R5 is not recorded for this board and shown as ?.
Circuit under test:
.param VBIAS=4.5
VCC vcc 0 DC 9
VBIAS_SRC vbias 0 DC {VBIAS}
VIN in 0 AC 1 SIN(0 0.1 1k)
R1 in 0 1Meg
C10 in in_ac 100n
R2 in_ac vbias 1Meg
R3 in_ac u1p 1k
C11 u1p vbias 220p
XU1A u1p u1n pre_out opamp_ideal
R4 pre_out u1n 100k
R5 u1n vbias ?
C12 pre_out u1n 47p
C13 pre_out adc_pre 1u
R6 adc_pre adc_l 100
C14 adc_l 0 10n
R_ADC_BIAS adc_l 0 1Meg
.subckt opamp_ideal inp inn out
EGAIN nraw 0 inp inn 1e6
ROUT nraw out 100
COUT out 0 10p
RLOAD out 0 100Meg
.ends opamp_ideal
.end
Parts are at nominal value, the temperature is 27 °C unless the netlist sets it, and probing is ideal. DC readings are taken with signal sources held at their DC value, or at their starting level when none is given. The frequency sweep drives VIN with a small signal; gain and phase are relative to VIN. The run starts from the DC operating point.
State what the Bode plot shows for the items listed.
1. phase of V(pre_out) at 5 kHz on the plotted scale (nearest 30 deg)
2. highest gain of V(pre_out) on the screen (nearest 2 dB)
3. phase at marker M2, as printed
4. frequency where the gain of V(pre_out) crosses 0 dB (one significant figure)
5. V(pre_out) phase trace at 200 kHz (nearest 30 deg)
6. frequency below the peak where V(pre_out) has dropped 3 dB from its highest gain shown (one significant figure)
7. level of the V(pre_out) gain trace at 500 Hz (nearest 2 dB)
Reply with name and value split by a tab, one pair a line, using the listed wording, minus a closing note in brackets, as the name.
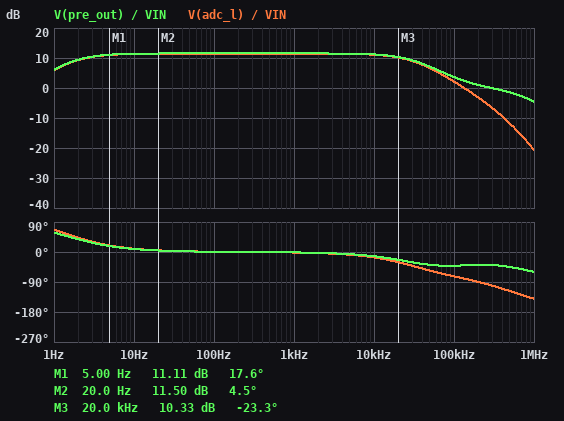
phase of V(pre_out) at 5 kHz on the plotted scale	0 deg
highest gain of V(pre_out) on the screen	12 dB
phase at marker M2, as printed	4.5 deg
frequency where the gain of V(pre_out) crosses 0 dB	300 kHz
V(pre_out) phase trace at 200 kHz	-30 deg
frequency below the peak where V(pre_out) has dropped 3 dB from its highest gain shown	2 Hz
level of the V(pre_out) gain trace at 500 Hz	12 dB
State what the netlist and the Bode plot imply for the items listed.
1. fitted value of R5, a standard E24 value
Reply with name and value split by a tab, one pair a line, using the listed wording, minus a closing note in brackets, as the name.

fitted value of R5, a standard E24 value	36 kΩ
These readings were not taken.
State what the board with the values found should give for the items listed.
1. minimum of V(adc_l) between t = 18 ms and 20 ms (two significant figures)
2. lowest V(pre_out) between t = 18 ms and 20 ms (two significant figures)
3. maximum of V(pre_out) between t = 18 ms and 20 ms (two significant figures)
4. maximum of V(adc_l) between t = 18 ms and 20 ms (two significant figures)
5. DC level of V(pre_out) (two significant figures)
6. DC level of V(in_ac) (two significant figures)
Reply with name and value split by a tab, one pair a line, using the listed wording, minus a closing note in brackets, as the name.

minimum of V(adc_l) between t = 18 ms and 20 ms	-370 mV
lowest V(pre_out) between t = 18 ms and 20 ms	4.1 V
maximum of V(pre_out) between t = 18 ms and 20 ms	4.9 V
maximum of V(adc_l) between t = 18 ms and 20 ms	370 mV
DC level of V(pre_out)	4.5 V
DC level of V(in_ac)	4.5 V
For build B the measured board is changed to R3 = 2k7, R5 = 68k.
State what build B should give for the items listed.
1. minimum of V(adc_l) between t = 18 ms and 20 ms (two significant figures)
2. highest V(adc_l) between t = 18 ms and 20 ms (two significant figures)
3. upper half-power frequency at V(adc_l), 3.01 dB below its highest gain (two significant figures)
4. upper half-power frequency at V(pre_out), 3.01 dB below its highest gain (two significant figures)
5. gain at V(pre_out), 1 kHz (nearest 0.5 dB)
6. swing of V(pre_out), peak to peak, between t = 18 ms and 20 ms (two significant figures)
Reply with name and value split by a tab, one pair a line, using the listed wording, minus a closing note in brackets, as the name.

minimum of V(adc_l) between t = 18 ms and 20 ms	-240 mV
highest V(adc_l) between t = 18 ms and 20 ms	240 mV
upper half-power frequency at V(adc_l), 3.01 dB below its highest gain	38 kHz
upper half-power frequency at V(pre_out), 3.01 dB below its highest gain	40 kHz
gain at V(pre_out), 1 kHz	8.0 dB
swing of V(pre_out), peak to peak, between t = 18 ms and 20 ms	490 mV
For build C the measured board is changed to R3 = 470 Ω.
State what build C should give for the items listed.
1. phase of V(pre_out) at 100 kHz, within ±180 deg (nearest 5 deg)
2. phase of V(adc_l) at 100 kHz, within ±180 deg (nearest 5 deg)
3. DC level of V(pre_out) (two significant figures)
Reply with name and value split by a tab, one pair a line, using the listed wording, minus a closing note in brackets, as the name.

phase of V(pre_out) at 100 kHz, within ±180 deg	-35 deg
phase of V(adc_l) at 100 kHz, within ±180 deg	-70 deg
DC level of V(pre_out)	4.5 V
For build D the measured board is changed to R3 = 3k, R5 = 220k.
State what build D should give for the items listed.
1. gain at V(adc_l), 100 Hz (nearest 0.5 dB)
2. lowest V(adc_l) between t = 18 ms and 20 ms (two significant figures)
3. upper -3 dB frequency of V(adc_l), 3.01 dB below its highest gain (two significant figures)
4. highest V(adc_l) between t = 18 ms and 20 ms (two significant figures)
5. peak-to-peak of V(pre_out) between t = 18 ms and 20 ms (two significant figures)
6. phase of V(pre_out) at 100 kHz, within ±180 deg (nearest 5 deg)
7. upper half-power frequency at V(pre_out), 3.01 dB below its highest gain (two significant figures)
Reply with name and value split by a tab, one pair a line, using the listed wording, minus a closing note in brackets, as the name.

gain at V(adc_l), 100 Hz	3.0 dB
lowest V(adc_l) between t = 18 ms and 20 ms	-140 mV
upper -3 dB frequency of V(adc_l), 3.01 dB below its highest gain	59 kHz
highest V(adc_l) between t = 18 ms and 20 ms	140 mV
peak-to-peak of V(pre_out) between t = 18 ms and 20 ms	290 mV
phase of V(pre_out) at 100 kHz, within ±180 deg	-30 deg
upper half-power frequency at V(pre_out), 3.01 dB below its highest gain	79 kHz
